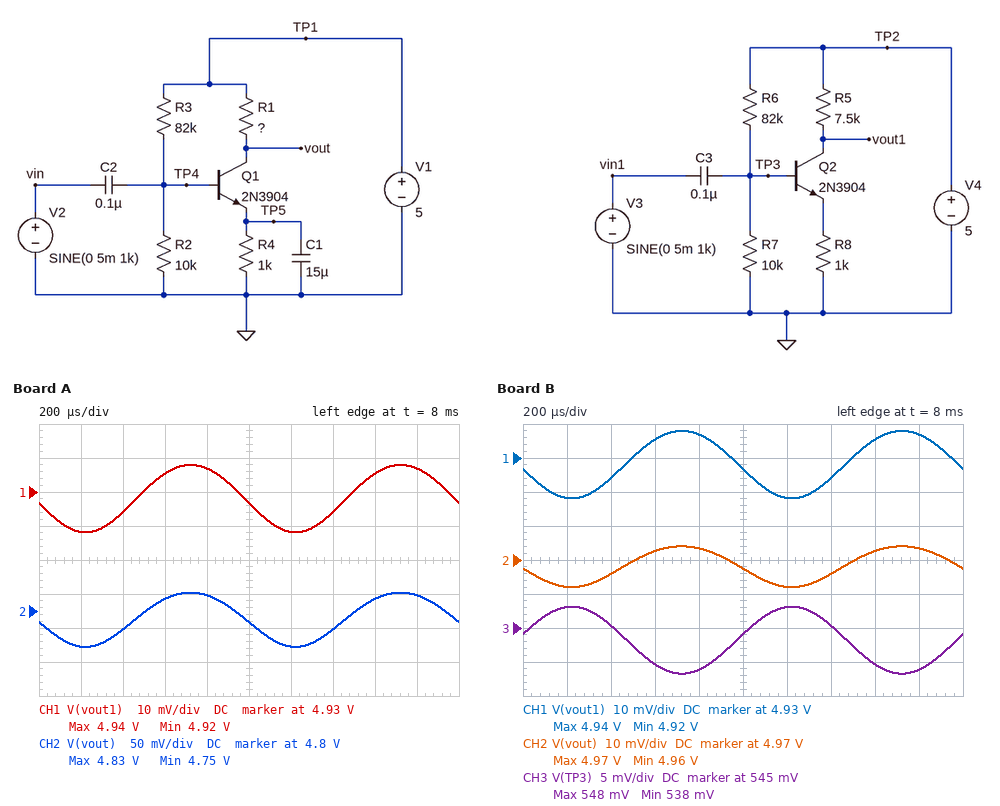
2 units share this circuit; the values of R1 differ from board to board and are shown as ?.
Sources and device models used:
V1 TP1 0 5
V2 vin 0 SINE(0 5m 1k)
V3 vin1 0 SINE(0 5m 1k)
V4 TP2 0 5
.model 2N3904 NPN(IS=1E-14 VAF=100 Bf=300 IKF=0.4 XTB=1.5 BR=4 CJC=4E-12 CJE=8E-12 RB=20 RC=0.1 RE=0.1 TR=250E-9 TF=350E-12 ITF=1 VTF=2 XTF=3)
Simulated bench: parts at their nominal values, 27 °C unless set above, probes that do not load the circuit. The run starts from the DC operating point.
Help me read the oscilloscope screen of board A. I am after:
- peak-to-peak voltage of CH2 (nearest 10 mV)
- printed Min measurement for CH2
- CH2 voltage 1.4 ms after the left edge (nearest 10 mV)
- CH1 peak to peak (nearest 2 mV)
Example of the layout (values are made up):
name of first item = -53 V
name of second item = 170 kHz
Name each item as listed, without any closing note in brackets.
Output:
peak-to-peak voltage of CH2 = 80 mV
printed Min measurement for CH2 = 4.75 V
CH2 voltage 1.4 ms after the left edge = 4.77 V
CH1 peak to peak = 20 mV
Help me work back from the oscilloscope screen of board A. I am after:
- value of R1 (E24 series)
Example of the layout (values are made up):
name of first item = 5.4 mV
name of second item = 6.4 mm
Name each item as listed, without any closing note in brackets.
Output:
value of R1 = 22 kΩ
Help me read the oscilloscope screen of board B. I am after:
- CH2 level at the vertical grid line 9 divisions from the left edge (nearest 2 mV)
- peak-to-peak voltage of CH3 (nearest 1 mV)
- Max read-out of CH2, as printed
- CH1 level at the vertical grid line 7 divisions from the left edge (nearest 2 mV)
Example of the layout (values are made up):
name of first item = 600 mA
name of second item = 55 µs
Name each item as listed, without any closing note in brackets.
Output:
CH2 level at the vertical grid line 9 divisions from the left edge = 4.974 V
peak-to-peak voltage of CH3 = 10 mV
Max read-out of CH2, as printed = 4.97 V
CH1 level at the vertical grid line 7 divisions from the left edge = 4.924 V
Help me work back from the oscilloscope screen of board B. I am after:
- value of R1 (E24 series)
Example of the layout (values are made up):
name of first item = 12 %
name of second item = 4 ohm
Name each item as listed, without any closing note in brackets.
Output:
value of R1 = 3.3 kΩ
